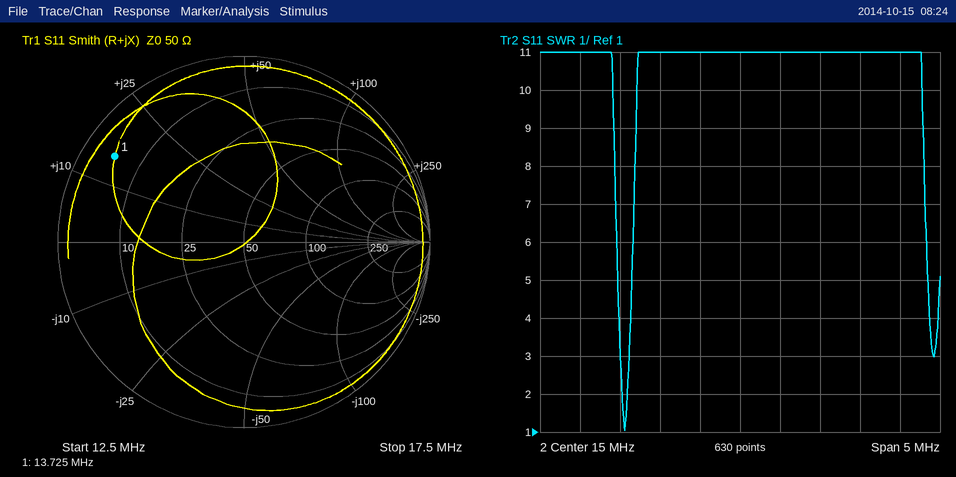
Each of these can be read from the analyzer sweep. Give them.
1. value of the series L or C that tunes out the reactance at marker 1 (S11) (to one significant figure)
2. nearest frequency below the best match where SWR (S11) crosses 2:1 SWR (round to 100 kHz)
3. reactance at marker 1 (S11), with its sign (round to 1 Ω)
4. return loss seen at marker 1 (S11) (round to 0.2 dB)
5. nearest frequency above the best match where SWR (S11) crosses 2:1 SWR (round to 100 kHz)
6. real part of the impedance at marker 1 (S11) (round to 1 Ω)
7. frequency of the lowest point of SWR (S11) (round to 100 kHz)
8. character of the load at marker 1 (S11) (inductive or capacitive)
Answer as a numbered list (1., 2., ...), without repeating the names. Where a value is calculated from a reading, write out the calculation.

1. C = 1/(2π × 13.725 MHz × 15 Ω) ≈ 773 pF, so 800 pF to one significant figure
2. 13.5 MHz
3. +15 Ω
4. 1.6 dB
5. 13.6 MHz
6. 5 Ω
7. 13.6 MHz
8. inductive
